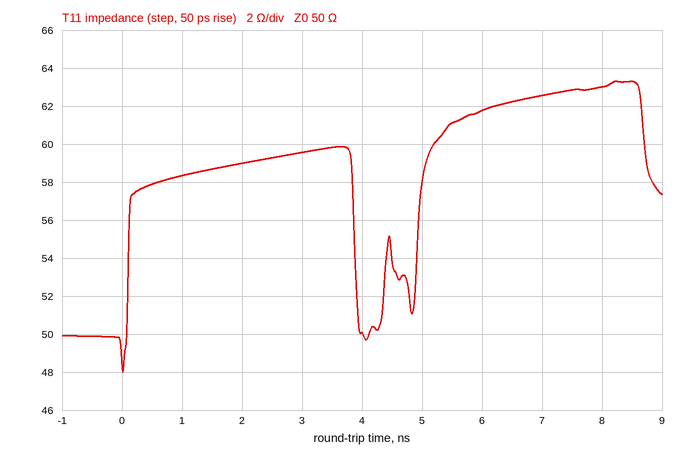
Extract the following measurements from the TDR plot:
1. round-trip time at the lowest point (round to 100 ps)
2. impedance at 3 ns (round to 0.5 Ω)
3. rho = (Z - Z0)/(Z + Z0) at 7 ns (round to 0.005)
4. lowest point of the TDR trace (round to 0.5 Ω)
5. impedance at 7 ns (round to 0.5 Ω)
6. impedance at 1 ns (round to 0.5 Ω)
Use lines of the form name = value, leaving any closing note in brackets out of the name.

round-trip time at the lowest point = 0.0 ns
impedance at 3 ns = 59.5 Ω
rho = (Z - Z0)/(Z + Z0) at 7 ns = +0.110
lowest point of the TDR trace = 48.0 Ω
impedance at 7 ns = 62.5 Ω
impedance at 1 ns = 58.5 Ω
